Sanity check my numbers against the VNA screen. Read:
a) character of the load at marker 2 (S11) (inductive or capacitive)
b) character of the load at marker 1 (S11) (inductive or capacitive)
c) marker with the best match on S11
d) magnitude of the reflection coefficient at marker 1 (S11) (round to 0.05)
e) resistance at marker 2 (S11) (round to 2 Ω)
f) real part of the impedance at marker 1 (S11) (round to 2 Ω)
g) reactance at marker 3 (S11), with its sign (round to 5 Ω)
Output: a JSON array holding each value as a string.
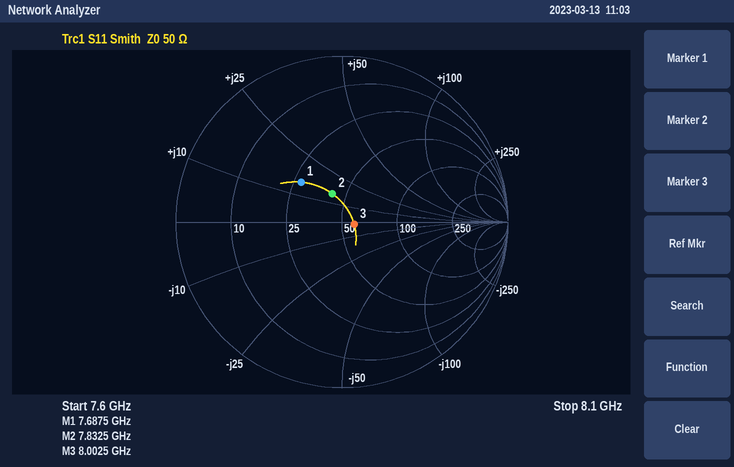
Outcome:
["inductive", "inductive", "marker 3", "0.35", "42 Ω", "28 Ω", "0 Ω"]
